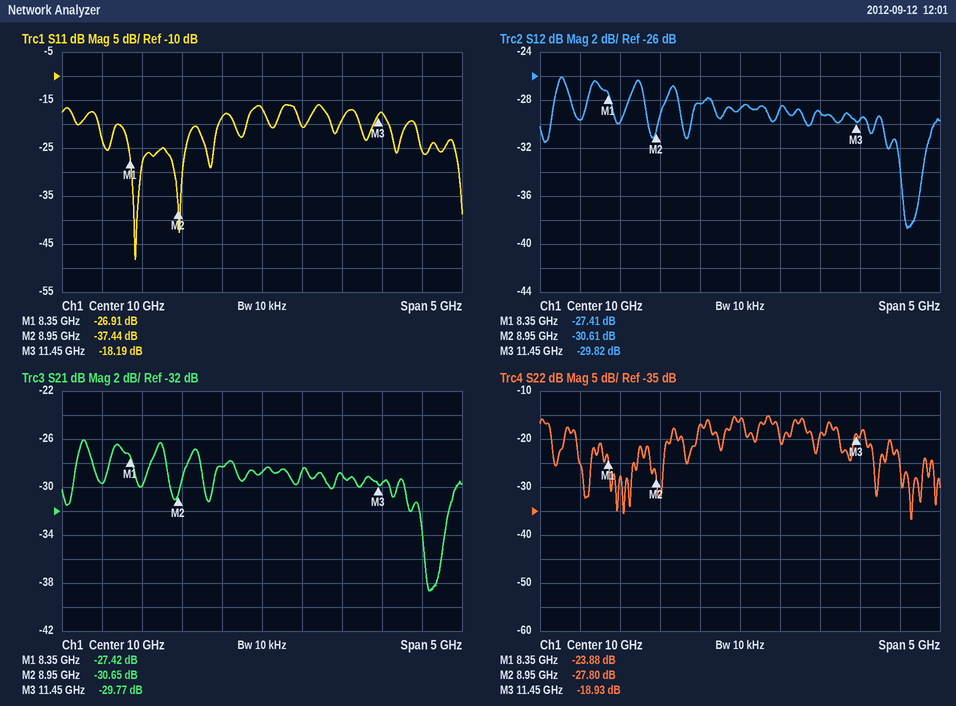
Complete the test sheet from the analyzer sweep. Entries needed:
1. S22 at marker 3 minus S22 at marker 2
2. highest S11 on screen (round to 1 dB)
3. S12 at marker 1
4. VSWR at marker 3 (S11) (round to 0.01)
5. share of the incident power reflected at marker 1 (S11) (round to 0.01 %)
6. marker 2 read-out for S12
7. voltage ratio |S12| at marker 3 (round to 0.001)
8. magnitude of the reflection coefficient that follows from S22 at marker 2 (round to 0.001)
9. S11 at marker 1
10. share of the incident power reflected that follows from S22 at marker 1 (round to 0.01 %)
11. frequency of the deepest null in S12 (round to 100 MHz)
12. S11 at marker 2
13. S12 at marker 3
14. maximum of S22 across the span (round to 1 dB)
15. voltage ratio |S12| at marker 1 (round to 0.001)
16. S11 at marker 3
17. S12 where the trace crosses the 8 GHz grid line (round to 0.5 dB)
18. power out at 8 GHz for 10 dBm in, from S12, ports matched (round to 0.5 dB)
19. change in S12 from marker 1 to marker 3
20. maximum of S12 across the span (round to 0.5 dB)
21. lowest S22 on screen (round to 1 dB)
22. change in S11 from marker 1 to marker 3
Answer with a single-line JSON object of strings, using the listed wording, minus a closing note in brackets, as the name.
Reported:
{"S22 at marker 3 minus S22 at marker 2": "8.87 dB", "highest S11 on screen": "-16 dB", "S12 at marker 1": "-27.41 dB", "VSWR at marker 3 (S11)": "1.28", "share of the incident power reflected at marker 1 (S11)": "0.20 %", "marker 2 read-out for S12": "-30.61 dB", "voltage ratio |S12| at marker 3": "0.032", "magnitude of the reflection coefficient that follows from S22 at marker 2": "0.041", "S11 at marker 1": "-26.91 dB", "share of the incident power reflected that follows from S22 at marker 1": "0.41 %", "frequency of the deepest null in S12": "12.1 GHz", "S11 at marker 2": "-37.44 dB", "S12 at marker 3": "-29.82 dB", "maximum of S22 across the span": "-15 dB", "voltage ratio |S12| at marker 1": "0.043", "S11 at marker 3": "-18.19 dB", "S12 where the trace crosses the 8 GHz grid line": "-29.5 dB", "power out at 8 GHz for 10 dBm in, from S12, ports matched": "-19.5 dBm", "change in S12 from marker 1 to marker 3": "-2.41 dB", "maximum of S12 across the span": "-26.0 dB", "lowest S22 on screen": "-37 dB", "change in S11 from marker 1 to marker 3": "8.72 dB"}
